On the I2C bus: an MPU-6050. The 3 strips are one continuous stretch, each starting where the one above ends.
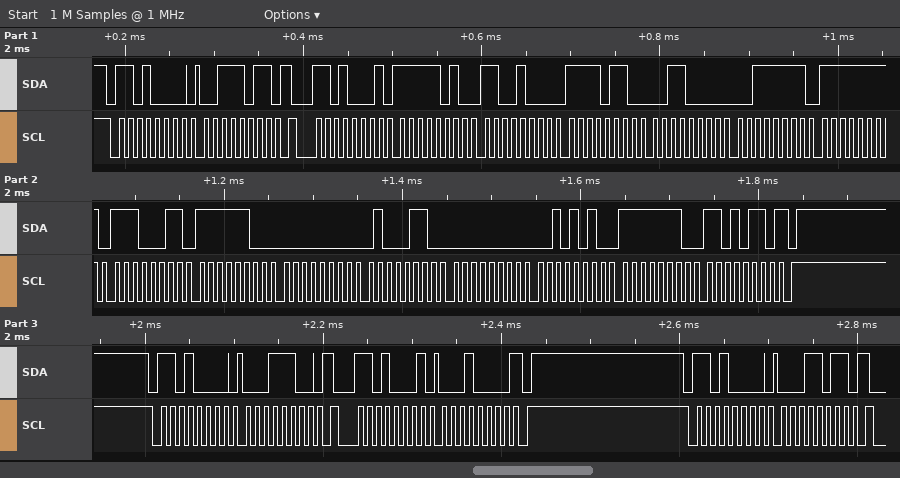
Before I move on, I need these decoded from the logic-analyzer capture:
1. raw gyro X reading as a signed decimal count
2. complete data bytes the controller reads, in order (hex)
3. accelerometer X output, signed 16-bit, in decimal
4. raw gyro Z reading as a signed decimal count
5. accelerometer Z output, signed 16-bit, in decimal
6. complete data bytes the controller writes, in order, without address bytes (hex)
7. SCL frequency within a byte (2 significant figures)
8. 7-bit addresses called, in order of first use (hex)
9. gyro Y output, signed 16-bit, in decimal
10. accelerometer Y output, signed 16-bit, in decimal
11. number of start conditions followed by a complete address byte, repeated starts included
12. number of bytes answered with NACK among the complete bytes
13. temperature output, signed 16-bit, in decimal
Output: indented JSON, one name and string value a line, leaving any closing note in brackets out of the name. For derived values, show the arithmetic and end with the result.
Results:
{
  "raw gyro X reading as a signed decimal count": "0x0046 = 70",
  "complete data bytes the controller reads, in order": "FA C8 F6 30 3F FF E3 FC 00 46 00 2A FE D6 10",
  "accelerometer X output, signed 16-bit, in decimal": "0xFAC8 = -1336",
  "raw gyro Z reading as a signed decimal count": "0xFED6 = -298",
  "accelerometer Z output, signed 16-bit, in decimal": "0x3FFF = 16383",
  "complete data bytes the controller writes, in order, without address bytes": "3B 1C 1B",
  "SCL frequency within a byte": "100 kHz",
  "7-bit addresses called, in order of first use": "0x68",
  "gyro Y output, signed 16-bit, in decimal": "0x002A = 42",
  "accelerometer Y output, signed 16-bit, in decimal": "0xF630 = -2512",
  "number of start conditions followed by a complete address byte, repeated starts included": "5",
  "number of bytes answered with NACK among the complete bytes": "2",
  "temperature output, signed 16-bit, in decimal": "0xE3FC = -7172"
}
